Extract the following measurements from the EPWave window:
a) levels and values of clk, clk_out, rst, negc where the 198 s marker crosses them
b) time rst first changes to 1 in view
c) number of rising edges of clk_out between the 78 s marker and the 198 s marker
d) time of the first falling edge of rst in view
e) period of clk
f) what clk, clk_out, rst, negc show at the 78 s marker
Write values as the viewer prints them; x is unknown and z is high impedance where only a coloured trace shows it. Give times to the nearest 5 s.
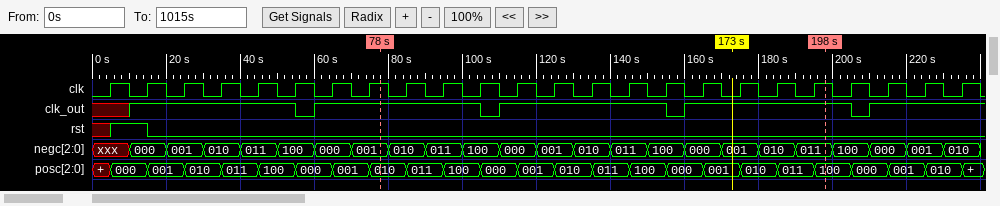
clk=1, clk_out=1, rst=0, negc=011
5 s
2
15 s
10 s
clk=1, clk_out=1, rst=0, negc=001
